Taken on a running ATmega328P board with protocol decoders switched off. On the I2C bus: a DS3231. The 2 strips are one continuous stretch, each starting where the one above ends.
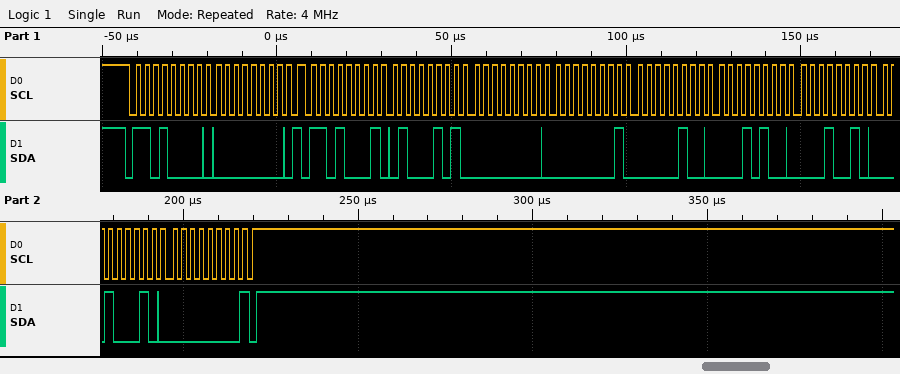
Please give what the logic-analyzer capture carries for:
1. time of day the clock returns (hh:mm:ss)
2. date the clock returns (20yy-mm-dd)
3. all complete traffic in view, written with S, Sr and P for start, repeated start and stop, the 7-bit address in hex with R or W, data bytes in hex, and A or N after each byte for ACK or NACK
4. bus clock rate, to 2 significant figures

01:00:45
2022-12-14
S 68W A 00 A Sr 68R A 45 A 00 A 01 A 04 A 14 A 12 A 22 A 00 N P
400 kHz
